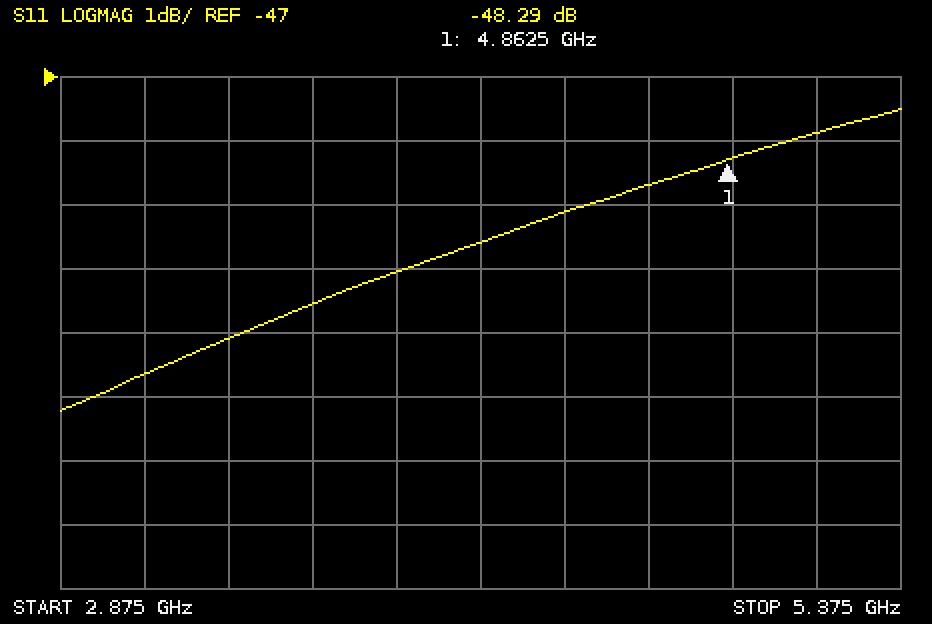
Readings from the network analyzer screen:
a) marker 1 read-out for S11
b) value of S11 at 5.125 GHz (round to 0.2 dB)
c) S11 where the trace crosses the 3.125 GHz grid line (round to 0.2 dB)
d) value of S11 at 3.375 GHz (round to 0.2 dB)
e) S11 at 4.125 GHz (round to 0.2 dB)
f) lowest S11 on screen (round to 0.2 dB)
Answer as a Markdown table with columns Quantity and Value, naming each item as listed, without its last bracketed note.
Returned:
| Quantity | Value |
|---|---|
| marker 1 read-out for S11 | -48.29 dB |
| value of S11 at 5.125 GHz | -47.8 dB |
| S11 where the trace crosses the 3.125 GHz grid line | -51.6 dB |
| value of S11 at 3.375 GHz | -51.0 dB |
| S11 at 4.125 GHz | -49.6 dB |
| lowest S11 on screen | -52.2 dB |
